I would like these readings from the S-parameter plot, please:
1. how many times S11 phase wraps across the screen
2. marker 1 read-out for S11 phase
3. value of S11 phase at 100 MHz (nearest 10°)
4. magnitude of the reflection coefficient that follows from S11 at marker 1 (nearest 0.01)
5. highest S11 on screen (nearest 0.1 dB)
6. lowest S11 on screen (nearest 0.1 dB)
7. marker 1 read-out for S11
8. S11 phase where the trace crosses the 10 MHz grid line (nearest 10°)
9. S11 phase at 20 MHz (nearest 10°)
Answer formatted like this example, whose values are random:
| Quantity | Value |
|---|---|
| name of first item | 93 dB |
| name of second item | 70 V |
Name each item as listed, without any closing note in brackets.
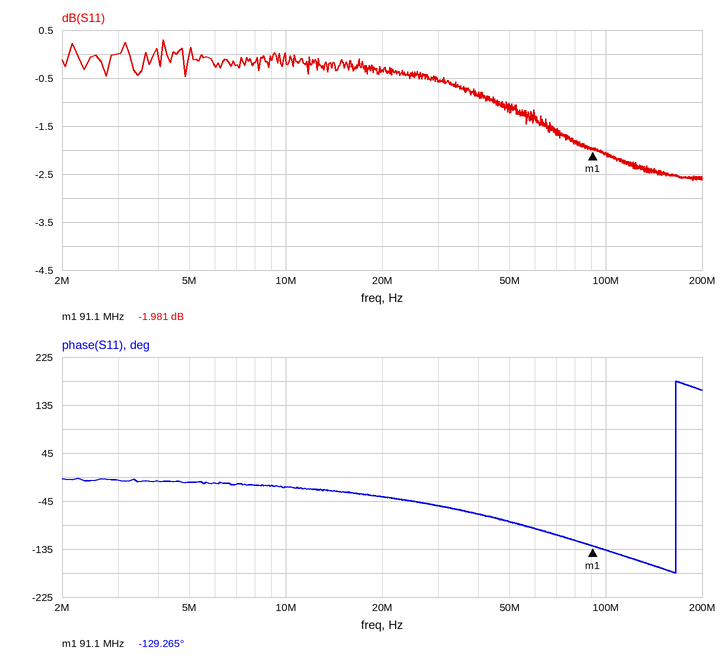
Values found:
| Quantity | Value |
|---|---|
| how many times S11 phase wraps across the screen | 1 |
| marker 1 read-out for S11 phase | -129.265° |
| value of S11 phase at 100 MHz | -140° |
| magnitude of the reflection coefficient that follows from S11 at marker 1 | 0.80 |
| highest S11 on screen | 0.3 dB |
| lowest S11 on screen | -2.6 dB |
| marker 1 read-out for S11 | -1.981 dB |
| S11 phase where the trace crosses the 10 MHz grid line | -20° |
| S11 phase at 20 MHz | -40° |
